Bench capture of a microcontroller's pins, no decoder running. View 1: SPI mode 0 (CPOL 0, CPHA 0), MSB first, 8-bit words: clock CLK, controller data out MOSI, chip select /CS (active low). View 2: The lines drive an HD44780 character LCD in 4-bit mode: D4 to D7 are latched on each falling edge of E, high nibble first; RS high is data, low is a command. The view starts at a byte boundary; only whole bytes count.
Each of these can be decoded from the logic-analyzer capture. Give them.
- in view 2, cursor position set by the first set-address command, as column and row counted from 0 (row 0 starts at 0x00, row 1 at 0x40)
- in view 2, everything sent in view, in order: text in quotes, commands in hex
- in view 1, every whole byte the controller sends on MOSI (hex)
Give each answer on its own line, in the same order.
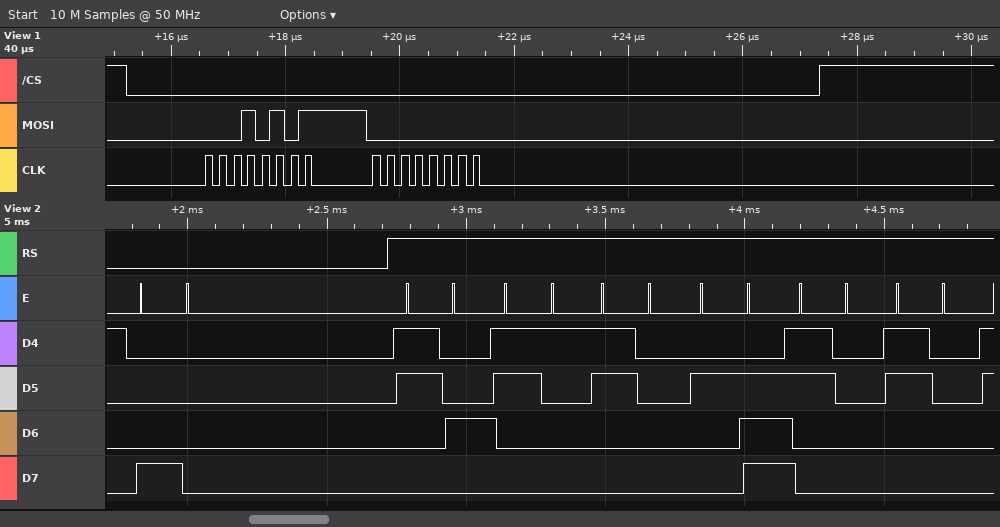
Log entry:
column 0, row 0
0x80 "410.00"
15 00
